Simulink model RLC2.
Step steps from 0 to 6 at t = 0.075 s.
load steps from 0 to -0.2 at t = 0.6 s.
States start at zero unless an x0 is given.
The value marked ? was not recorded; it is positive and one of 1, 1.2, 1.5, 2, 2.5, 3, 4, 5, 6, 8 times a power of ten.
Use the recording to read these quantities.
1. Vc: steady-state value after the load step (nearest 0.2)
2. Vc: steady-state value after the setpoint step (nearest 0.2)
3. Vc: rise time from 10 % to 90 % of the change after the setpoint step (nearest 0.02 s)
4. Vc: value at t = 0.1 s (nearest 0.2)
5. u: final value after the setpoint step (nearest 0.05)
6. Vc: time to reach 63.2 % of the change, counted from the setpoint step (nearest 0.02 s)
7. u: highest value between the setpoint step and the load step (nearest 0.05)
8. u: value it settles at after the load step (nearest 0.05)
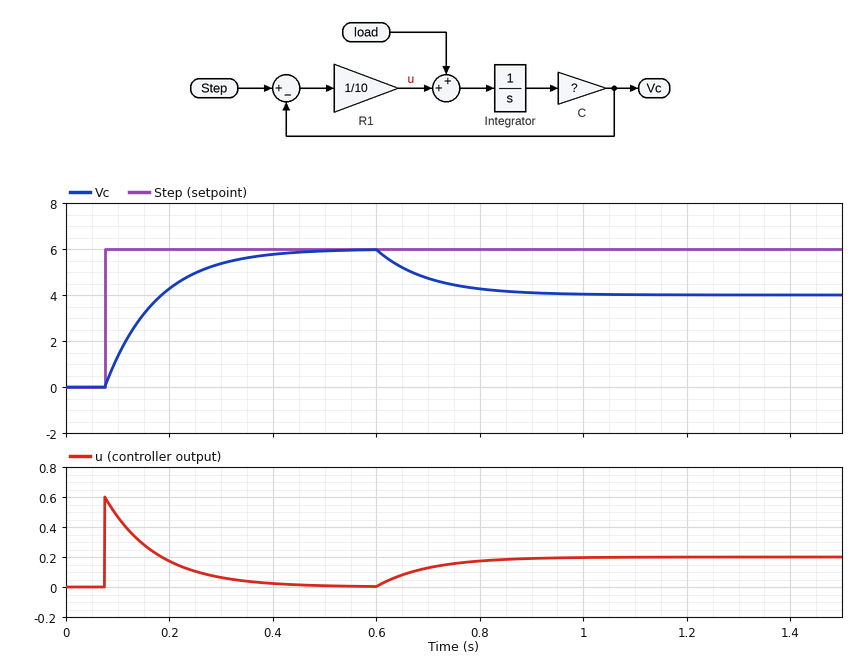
4.0
6.0
0.22 s
1.4
0.00
0.10 s
0.60
0.20
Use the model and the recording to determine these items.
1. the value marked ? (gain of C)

100
